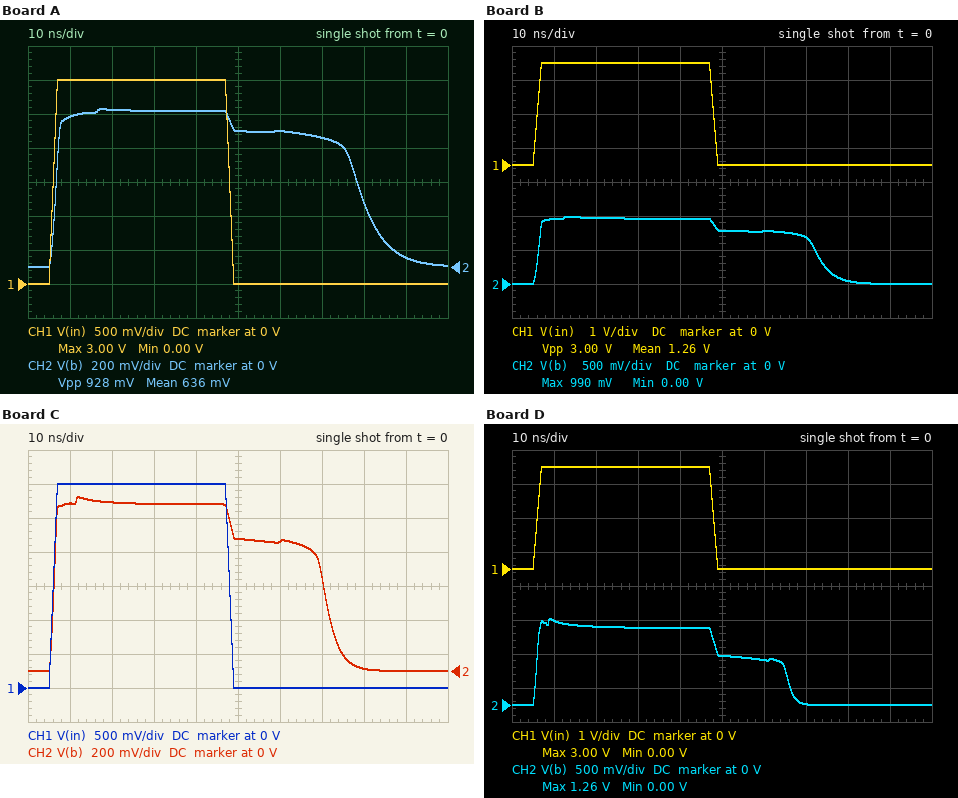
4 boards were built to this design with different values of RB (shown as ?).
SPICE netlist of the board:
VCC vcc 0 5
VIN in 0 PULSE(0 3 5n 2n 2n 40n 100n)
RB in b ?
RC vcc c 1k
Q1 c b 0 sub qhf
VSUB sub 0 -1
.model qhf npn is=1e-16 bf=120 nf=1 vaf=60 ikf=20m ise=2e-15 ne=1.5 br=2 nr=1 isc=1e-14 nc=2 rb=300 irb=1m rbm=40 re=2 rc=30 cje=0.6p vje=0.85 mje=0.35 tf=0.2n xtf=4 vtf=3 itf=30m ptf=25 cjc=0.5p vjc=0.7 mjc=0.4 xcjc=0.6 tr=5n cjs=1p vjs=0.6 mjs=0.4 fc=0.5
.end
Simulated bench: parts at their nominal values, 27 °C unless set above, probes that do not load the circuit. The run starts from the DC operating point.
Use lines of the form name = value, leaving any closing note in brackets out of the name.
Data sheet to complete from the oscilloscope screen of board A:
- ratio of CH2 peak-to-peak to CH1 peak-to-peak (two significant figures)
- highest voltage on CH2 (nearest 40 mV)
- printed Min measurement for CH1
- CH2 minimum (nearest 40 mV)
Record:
ratio of CH2 peak-to-peak to CH1 peak-to-peak = 0.31
highest voltage on CH2 = 920 mV
printed Min measurement for CH1 = 0.00 V
CH2 minimum = 0 V
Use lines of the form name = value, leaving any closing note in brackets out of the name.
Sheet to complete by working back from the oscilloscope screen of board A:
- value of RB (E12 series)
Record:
value of RB = 5.6 kΩ
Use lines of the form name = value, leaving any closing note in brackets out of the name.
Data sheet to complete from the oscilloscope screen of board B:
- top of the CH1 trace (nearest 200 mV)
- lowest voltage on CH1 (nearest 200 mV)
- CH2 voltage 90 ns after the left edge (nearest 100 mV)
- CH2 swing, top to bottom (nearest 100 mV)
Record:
top of the CH1 trace = 3.0 V
lowest voltage on CH1 = 0 V
CH2 voltage 90 ns after the left edge = 0 V
CH2 swing, top to bottom = 1.0 V
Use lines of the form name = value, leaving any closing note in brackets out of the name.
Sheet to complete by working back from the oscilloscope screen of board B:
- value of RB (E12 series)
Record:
value of RB = 3.3 kΩ
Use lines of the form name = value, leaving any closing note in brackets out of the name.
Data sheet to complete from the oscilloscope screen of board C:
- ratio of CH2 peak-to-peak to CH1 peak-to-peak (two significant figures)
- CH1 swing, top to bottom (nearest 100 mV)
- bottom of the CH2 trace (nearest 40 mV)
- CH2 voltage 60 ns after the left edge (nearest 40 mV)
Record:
ratio of CH2 peak-to-peak to CH1 peak-to-peak = 0.34
CH1 swing, top to bottom = 3.0 V
bottom of the CH2 trace = 0 V
CH2 voltage 60 ns after the left edge = 760 mV
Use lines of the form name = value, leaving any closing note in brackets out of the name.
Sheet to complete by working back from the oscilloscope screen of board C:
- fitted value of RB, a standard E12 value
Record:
fitted value of RB, a standard E12 value = 2.7 kΩ
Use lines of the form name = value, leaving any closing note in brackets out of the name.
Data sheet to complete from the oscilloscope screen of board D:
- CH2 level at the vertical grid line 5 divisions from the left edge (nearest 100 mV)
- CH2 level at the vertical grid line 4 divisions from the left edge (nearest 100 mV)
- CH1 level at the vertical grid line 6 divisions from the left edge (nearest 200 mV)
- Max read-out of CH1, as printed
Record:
CH2 level at the vertical grid line 5 divisions from the left edge = 700 mV
CH2 level at the vertical grid line 4 divisions from the left edge = 1.1 V
CH1 level at the vertical grid line 6 divisions from the left edge = 0 V
Max read-out of CH1, as printed = 3.00 V
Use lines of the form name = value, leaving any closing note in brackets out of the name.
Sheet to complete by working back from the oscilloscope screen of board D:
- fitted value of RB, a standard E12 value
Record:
fitted value of RB, a standard E12 value = 1 kΩ
